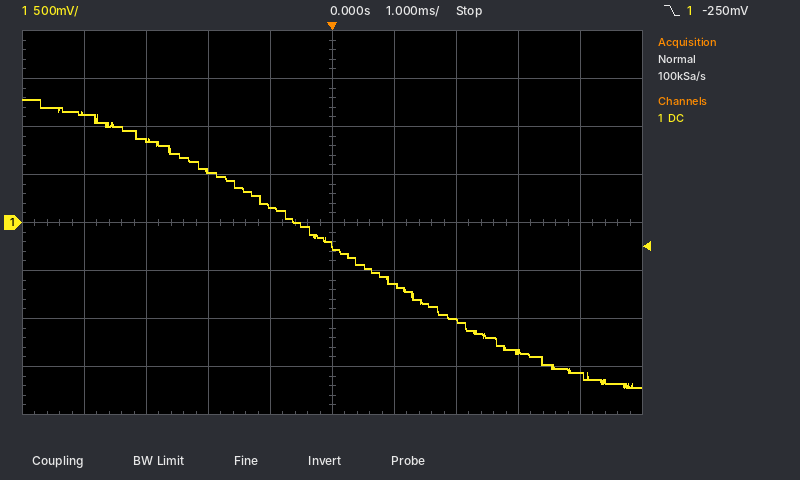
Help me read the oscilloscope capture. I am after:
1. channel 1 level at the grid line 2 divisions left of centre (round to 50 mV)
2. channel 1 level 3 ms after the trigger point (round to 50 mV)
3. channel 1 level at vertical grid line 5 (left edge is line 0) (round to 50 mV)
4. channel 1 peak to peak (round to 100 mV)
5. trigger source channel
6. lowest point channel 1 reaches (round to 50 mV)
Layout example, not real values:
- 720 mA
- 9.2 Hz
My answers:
- 550 mV
- -1.35 V
- -250 mV
- 3.00 V
- channel 1
- -1.70 V
